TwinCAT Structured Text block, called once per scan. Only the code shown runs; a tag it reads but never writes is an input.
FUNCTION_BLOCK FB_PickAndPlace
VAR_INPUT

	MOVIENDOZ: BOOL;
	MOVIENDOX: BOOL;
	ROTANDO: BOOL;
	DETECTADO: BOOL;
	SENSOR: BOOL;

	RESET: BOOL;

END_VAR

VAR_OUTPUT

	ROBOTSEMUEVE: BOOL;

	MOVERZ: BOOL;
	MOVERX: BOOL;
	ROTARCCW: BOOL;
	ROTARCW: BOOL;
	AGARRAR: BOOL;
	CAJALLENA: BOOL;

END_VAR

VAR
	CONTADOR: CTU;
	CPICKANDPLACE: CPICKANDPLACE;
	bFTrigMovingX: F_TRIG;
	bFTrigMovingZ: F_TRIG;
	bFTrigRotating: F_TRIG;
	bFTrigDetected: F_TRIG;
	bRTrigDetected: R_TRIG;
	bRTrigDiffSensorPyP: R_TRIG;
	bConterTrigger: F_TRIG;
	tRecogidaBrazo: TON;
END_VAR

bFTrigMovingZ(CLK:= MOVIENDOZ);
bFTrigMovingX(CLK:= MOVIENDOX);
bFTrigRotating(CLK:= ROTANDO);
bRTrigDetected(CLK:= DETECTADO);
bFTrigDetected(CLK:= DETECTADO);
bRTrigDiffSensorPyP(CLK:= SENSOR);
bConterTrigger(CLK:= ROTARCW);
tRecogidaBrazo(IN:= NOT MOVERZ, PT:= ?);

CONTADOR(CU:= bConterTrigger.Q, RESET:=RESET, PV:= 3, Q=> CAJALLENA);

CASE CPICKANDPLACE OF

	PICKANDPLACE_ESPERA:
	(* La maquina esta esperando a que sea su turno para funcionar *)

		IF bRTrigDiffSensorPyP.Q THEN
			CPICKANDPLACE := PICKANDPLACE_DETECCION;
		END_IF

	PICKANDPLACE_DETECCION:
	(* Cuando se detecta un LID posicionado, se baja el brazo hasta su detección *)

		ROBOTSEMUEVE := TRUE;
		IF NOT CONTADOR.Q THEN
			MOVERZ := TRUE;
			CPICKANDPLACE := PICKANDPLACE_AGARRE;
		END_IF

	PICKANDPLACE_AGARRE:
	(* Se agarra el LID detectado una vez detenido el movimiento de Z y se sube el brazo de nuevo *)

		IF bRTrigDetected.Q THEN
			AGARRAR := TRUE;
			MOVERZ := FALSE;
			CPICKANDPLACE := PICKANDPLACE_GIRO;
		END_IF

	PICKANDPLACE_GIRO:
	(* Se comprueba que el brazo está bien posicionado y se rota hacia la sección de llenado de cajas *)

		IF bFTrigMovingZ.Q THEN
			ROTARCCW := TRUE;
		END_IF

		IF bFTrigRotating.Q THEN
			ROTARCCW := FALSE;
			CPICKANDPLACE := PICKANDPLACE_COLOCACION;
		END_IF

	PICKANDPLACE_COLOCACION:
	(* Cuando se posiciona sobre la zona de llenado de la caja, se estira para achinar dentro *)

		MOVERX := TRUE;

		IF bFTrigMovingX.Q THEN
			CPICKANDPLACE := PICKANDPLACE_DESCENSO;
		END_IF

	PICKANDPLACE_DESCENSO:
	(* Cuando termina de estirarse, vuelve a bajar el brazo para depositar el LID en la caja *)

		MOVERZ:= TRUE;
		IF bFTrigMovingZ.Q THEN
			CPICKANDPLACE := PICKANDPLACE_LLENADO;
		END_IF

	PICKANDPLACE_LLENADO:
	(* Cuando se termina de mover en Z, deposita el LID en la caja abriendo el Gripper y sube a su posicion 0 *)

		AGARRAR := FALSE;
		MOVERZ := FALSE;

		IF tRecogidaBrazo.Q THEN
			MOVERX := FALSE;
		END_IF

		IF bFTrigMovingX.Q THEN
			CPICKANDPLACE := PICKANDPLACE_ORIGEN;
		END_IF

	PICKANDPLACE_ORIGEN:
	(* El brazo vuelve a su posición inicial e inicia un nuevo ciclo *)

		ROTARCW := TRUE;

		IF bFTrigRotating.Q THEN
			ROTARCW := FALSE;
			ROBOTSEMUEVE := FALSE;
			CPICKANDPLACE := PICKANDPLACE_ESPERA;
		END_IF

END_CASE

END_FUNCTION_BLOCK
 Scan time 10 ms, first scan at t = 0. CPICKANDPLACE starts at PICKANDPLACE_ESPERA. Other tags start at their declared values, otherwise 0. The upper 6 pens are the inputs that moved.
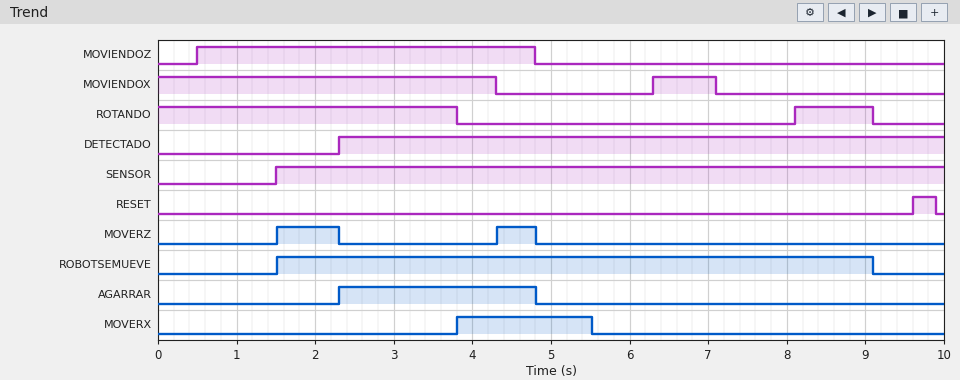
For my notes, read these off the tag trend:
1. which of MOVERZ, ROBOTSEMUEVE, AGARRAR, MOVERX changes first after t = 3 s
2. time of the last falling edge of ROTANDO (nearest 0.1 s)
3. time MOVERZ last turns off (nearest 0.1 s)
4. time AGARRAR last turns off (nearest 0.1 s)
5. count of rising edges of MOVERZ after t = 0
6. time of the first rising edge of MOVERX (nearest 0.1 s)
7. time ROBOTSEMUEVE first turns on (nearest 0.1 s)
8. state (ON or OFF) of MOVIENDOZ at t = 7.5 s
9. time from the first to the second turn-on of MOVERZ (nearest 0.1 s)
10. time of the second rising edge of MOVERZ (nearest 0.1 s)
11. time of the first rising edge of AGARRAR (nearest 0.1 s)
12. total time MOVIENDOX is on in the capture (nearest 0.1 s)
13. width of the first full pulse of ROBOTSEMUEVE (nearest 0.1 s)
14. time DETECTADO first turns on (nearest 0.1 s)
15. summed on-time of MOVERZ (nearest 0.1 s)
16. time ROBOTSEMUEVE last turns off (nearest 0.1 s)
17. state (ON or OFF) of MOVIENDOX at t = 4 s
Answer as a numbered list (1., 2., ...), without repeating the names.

1. MOVERX
2. 9.1 s
3. 4.8 s
4. 4.8 s
5. 2
6. 3.8 s
7. 1.5 s
8. OFF
9. 2.8 s
10. 4.3 s
11. 2.3 s
12. 5.1 s
13. 7.6 s
14. 2.3 s
15. 1.3 s
16. 9.1 s
17. ON
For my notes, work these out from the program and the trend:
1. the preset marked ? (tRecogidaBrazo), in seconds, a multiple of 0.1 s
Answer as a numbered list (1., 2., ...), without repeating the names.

1. 0.7 s
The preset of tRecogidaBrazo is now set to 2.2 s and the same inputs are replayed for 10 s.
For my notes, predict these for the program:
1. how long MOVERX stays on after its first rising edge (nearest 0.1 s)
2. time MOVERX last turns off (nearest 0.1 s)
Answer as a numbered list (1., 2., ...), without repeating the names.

1. 3.2 s
2. 7.0 s
